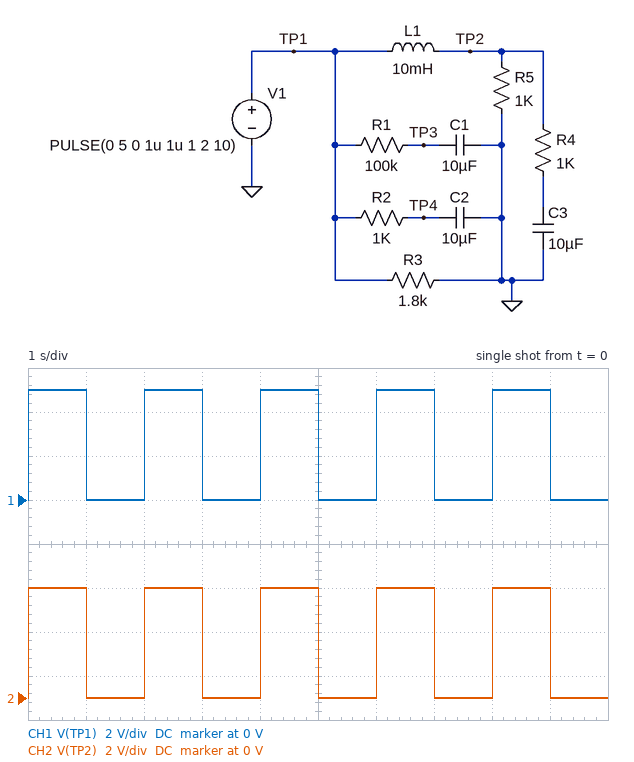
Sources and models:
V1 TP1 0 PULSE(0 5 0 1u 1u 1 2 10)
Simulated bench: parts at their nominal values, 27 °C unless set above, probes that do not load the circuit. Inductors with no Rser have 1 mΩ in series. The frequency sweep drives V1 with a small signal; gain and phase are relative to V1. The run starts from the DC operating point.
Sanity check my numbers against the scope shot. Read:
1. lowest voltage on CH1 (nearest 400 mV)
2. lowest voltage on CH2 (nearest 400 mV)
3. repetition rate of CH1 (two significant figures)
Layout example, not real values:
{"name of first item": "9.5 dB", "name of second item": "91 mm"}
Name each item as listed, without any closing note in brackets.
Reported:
{"lowest voltage on CH1": "0 V", "lowest voltage on CH2": "0 V", "repetition rate of CH1": "500 mHz"}
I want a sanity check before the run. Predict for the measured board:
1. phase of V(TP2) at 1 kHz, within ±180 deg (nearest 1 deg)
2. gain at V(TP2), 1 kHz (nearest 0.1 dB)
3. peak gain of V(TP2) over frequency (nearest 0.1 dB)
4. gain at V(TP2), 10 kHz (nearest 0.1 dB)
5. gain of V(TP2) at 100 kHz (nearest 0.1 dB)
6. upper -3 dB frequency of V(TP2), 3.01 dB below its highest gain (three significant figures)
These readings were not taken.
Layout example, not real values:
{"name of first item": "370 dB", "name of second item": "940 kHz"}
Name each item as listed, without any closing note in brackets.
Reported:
{"phase of V(TP2) at 1 kHz, within ±180 deg": "-7 deg", "gain at V(TP2), 1 kHz": "-0.1 dB", "peak gain of V(TP2) over frequency": "0 dB", "gain at V(TP2), 10 kHz": "-4.1 dB", "gain of V(TP2) at 100 kHz": "-22.0 dB", "upper -3 dB frequency of V(TP2), 3.01 dB below its highest gain": "7.95 kHz"}
